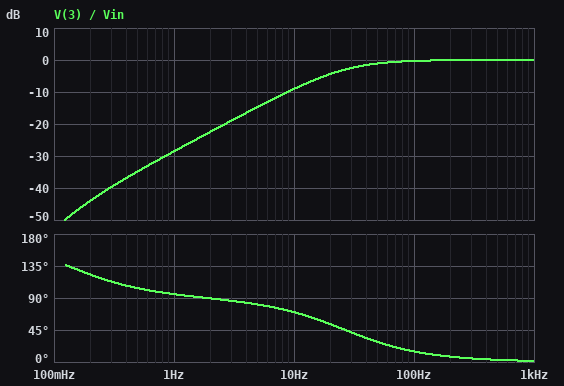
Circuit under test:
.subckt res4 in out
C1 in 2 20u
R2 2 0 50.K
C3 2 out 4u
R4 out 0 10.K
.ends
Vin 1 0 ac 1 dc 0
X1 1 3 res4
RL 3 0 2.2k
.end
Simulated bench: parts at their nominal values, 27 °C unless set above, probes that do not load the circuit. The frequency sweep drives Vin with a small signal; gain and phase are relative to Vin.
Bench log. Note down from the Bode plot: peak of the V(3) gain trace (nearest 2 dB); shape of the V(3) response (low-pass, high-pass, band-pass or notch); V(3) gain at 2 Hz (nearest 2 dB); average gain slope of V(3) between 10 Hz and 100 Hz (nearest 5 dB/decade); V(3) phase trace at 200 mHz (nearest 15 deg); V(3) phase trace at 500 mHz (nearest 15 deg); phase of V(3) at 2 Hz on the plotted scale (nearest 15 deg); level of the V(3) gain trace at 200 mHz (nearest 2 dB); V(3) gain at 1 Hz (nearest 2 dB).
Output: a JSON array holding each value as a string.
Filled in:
["0 dB", "high-pass", "-22 dB", "10 dB/decade", "120 deg", "105 deg", "90 deg", "-44 dB", "-28 dB"]
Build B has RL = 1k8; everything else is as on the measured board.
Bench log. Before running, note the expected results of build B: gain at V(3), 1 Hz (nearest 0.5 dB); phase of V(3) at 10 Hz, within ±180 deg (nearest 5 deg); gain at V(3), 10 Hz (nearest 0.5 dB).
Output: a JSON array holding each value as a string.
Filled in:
["-30.0 dB", "75 deg", "-10.5 dB"]
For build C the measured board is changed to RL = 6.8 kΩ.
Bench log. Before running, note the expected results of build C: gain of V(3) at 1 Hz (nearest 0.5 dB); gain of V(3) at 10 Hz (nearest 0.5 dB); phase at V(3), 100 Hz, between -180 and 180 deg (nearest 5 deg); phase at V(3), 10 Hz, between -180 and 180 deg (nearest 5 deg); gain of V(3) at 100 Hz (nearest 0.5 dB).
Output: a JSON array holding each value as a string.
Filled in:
["-21.5 dB", "-4.0 dB", "5 deg", "50 deg", "0 dB"]
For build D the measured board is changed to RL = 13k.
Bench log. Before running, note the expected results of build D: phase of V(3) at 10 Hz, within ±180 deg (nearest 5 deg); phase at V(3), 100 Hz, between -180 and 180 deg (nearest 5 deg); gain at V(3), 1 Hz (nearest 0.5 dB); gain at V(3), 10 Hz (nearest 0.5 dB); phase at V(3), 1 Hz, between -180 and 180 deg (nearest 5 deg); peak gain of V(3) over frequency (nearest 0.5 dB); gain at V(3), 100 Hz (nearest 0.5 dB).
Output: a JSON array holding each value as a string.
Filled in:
["40 deg", "5 deg", "-18.5 dB", "-2.5 dB", "90 deg", "0 dB", "0 dB"]
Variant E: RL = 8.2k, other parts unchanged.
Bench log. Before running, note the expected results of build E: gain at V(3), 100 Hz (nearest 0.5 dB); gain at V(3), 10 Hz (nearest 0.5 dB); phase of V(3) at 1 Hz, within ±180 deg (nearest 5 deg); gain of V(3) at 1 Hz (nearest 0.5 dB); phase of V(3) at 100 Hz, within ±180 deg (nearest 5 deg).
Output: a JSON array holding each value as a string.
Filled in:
["0 dB", "-3.5 dB", "90 deg", "-20.5 dB", "5 deg"]
